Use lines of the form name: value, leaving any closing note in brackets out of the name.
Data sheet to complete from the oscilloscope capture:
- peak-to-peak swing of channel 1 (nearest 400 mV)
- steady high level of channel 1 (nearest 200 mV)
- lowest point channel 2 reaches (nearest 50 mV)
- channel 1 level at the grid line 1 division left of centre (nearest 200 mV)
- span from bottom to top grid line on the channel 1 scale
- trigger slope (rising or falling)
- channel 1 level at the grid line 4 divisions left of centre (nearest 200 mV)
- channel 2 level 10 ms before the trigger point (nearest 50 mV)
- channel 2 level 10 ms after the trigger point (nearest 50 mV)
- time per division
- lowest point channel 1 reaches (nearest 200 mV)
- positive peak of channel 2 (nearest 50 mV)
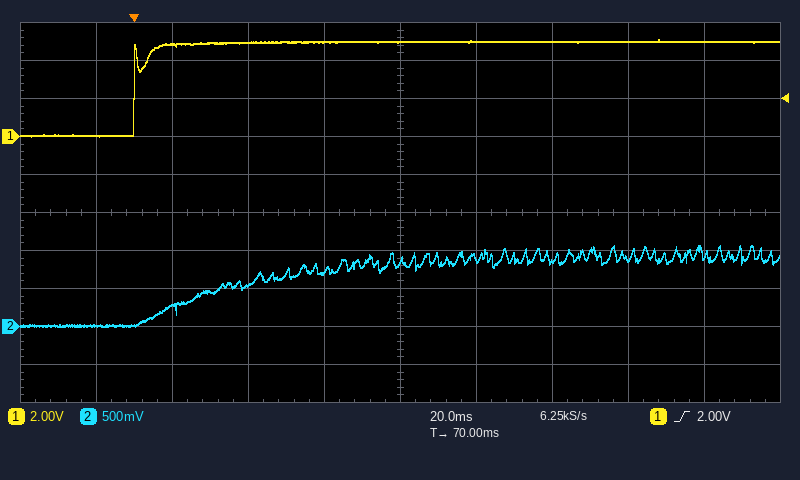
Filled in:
peak-to-peak swing of channel 1: 5.2 V
steady high level of channel 1: 5.0 V
lowest point channel 2 reaches: 0 mV
channel 1 level at the grid line 1 division left of centre: 5.0 V
span from bottom to top grid line on the channel 1 scale: 20 V
trigger slope: rising
channel 1 level at the grid line 4 divisions left of centre: 0.0 V
channel 2 level 10 ms before the trigger point: 0 mV
channel 2 level 10 ms after the trigger point: 250 mV
time per division: 20 ms
lowest point channel 1 reaches: 0.0 V
positive peak of channel 2: 1.05 V
